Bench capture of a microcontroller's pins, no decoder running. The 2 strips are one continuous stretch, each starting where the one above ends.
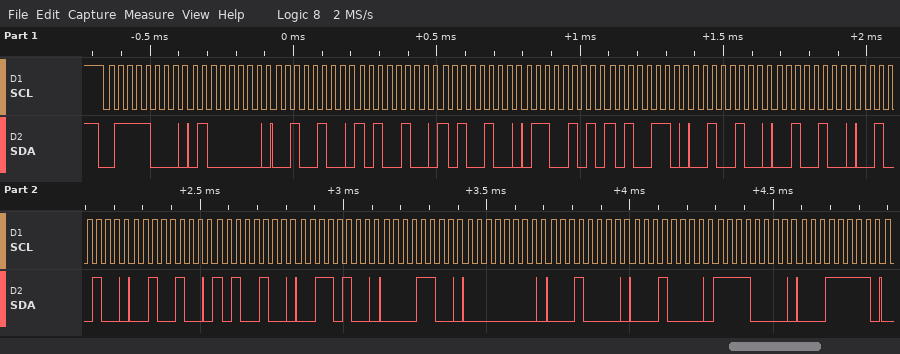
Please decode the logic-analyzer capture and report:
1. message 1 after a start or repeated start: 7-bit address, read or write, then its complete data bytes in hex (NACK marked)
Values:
0x3C write: 40 24 A4 A4 65 A6 24 24 24 24 A4 34 0C 00 10 10 F0 1F
